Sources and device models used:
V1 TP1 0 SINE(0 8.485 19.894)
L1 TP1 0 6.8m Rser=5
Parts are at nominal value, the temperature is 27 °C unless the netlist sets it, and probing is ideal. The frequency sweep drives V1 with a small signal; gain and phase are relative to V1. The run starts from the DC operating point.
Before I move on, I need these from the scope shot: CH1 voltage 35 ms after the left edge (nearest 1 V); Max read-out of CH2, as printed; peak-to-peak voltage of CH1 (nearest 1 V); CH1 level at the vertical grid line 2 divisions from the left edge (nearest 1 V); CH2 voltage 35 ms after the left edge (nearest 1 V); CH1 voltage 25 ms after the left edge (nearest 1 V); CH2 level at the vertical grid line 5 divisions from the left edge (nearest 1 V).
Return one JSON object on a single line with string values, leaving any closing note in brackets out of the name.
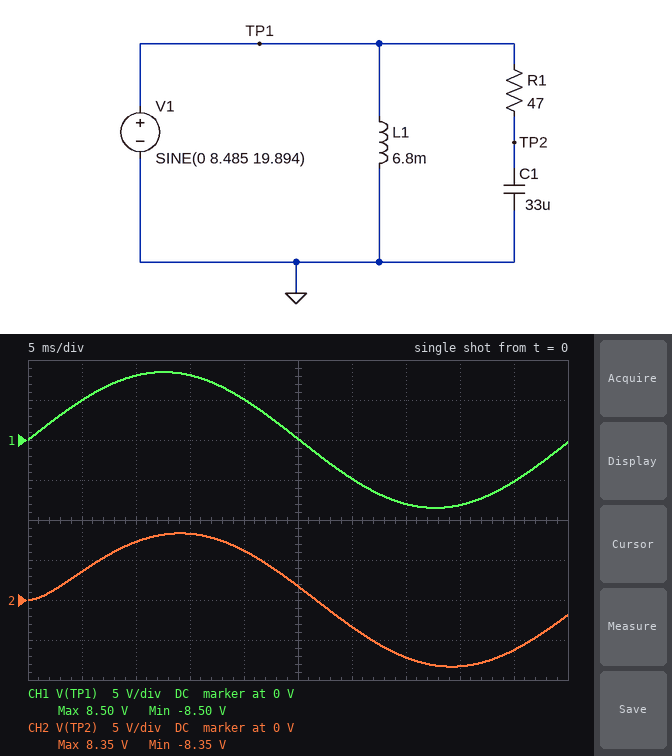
{"CH1 voltage 35 ms after the left edge": "-8 V", "Max read-out of CH2, as printed": "8.35 V", "peak-to-peak voltage of CH1": "17 V", "CH1 level at the vertical grid line 2 divisions from the left edge": "8 V", "CH2 voltage 35 ms after the left edge": "-7 V", "CH1 voltage 25 ms after the left edge": "0 V", "CH2 level at the vertical grid line 5 divisions from the left edge": "2 V"}
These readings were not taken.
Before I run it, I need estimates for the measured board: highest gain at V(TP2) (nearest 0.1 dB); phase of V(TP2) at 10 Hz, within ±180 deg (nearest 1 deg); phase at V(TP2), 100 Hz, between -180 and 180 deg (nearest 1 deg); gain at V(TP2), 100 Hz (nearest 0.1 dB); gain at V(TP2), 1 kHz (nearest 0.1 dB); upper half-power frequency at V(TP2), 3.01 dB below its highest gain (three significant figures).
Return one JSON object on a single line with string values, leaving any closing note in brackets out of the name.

{"highest gain at V(TP2)": "0 dB", "phase of V(TP2) at 10 Hz, within ±180 deg": "-6 deg", "phase at V(TP2), 100 Hz, between -180 and 180 deg": "-44 deg", "gain at V(TP2), 100 Hz": "-2.9 dB", "gain at V(TP2), 1 kHz": "-19.8 dB", "upper half-power frequency at V(TP2), 3.01 dB below its highest gain": "103 Hz"}
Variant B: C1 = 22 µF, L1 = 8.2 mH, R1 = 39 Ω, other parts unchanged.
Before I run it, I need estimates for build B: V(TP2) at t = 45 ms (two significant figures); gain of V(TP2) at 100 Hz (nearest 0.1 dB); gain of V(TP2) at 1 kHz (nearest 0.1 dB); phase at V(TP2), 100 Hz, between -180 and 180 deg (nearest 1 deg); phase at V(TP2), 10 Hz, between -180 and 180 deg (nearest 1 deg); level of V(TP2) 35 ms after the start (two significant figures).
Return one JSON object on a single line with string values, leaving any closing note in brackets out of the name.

{"V(TP2) at t = 45 ms": "-5.8 V", "gain of V(TP2) at 100 Hz": "-1.1 dB", "gain of V(TP2) at 1 kHz": "-14.8 dB", "phase at V(TP2), 100 Hz, between -180 and 180 deg": "-28 deg", "phase at V(TP2), 10 Hz, between -180 and 180 deg": "-3 deg", "level of V(TP2) 35 ms after the start": "-7.6 V"}
